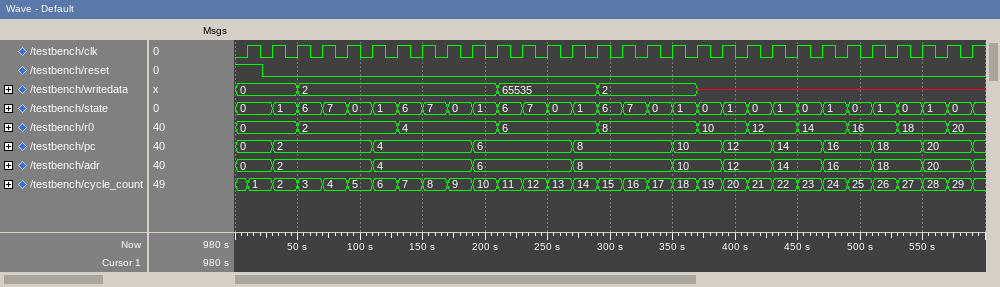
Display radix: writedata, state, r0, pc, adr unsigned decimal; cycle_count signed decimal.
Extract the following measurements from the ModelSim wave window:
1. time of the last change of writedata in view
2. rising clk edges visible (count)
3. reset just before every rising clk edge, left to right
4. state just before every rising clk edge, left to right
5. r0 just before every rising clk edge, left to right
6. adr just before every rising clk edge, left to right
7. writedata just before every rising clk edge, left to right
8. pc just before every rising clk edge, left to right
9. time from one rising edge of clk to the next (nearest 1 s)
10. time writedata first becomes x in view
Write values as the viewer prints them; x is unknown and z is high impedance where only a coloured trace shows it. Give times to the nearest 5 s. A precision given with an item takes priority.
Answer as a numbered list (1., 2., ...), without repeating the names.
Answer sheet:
1. 370 s
2. 30
3. 1 0 0 0 0 0 0 0 0 0 0 0 0 0 0 0 0 0 0 0 0 0 0 0 0 0 0 0 0 0
4. 0, 0, 1, 6, 7, 0, 1, 6, 7, 0, 1, 6, 7, 0, 1, 6, 7, 0, 1, 0, 1, 0, 1, 0, 1, 0, 1, 0, 1, 0
5. 0, 0, 0, 2, 2, 2, 2, 4, 4, 4, 4, 6, 6, 6, 6, 8, 8, 8, 8, 10, 10, 12, 12, 14, 14, 16, 16, 18, 18, 20
6. 0, 0, 2, 2, 2, 2, 4, 4, 4, 4, 6, 6, 6, 6, 8, 8, 8, 8, 10, 10, 12, 12, 14, 14, 16, 16, 18, 18, 20, 20
7. 0, 0, 0, 2, 2, 2, 2, 2, 2, 2, 2, 65535, 65535, 65535, 65535, 2, 2, 2, 2, x, x, x, x, x, x, x, x, x, x, x
8. 0, 0, 2, 2, 2, 2, 4, 4, 4, 4, 6, 6, 6, 6, 8, 8, 8, 8, 10, 10, 12, 12, 14, 14, 16, 16, 18, 18, 20, 20
9. 20 s
10. 370 s
